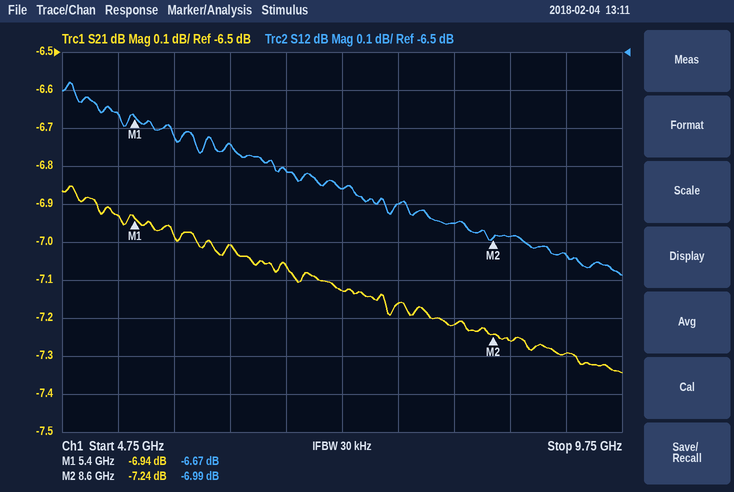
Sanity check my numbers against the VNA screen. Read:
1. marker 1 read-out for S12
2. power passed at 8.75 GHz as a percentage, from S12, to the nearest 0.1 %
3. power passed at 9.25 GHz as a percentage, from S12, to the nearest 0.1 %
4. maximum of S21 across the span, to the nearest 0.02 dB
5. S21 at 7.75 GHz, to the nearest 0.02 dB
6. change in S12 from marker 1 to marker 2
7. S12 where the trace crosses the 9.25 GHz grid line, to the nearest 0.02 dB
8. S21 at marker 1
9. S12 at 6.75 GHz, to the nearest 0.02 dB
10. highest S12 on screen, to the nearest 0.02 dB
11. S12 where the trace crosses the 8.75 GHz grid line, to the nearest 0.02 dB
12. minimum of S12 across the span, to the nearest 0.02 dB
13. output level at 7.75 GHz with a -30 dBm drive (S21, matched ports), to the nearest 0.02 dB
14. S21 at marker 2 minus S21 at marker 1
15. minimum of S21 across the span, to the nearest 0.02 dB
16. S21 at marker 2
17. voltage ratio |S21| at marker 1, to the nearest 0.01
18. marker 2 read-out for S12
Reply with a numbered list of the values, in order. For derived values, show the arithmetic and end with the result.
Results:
1. -6.67 dB
2. 10^(-6.98/10) ≈ 20.0 %
3. 10^(-7.04/10) ≈ 19.8 %
4. -6.86 dB
5. -7.16 dB
6. -6.99 − (-6.67) = -0.32 dB
7. -7.04 dB
8. -6.94 dB
9. -6.82 dB
10. -6.58 dB
11. -6.98 dB
12. -7.08 dB
13. -30 dBm + (-7.16 dB) = -37.16 dBm
14. -7.24 − (-6.94) = -0.30 dB
15. -7.34 dB
16. -7.24 dB
17. 10^(-6.94/20) ≈ 0.45
18. -6.99 dB
